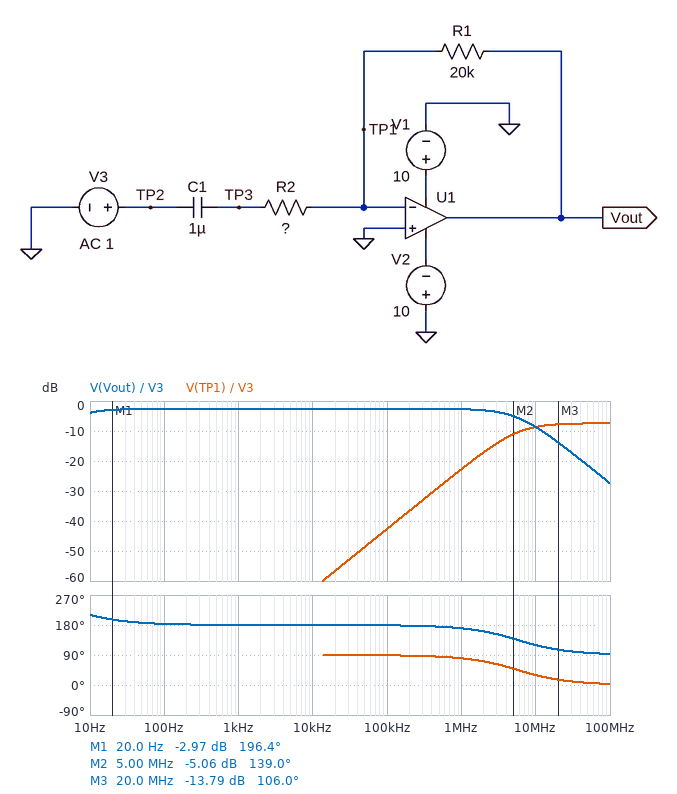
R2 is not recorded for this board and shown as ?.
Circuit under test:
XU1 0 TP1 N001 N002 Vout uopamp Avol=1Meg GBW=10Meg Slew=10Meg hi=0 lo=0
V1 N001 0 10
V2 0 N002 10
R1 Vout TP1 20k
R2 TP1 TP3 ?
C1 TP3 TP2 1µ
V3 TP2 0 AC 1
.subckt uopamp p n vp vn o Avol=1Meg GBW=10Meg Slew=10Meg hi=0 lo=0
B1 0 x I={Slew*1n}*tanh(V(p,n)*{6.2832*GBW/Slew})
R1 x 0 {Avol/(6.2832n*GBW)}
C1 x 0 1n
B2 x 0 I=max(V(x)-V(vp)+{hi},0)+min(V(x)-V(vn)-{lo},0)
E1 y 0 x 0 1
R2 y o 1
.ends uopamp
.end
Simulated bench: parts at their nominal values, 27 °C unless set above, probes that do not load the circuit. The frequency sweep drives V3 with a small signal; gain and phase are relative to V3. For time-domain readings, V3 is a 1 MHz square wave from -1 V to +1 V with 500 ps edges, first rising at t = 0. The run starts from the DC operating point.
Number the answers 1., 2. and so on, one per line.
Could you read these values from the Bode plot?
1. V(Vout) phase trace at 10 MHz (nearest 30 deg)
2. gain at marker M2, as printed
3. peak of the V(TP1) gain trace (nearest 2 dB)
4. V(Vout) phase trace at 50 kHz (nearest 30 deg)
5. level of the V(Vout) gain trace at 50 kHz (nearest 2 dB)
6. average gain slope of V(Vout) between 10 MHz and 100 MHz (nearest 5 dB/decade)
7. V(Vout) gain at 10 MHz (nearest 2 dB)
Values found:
1. 120 deg
2. -5.06 dB
3. -8 dB
4. 180 deg
5. -2 dB
6. -20 dB/decade
7. -8 dB
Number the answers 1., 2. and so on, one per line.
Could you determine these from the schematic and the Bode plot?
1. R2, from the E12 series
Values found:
1. 27 kΩ
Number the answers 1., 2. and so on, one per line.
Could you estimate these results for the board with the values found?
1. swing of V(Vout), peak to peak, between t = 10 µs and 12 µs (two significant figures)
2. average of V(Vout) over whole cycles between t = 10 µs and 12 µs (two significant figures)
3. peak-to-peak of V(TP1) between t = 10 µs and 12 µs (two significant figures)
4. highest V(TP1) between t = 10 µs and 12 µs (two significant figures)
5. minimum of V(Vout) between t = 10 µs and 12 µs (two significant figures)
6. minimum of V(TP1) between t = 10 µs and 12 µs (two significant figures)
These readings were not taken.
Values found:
1. 1.5 V
2. -740 mV
3. 1.7 V
4. 850 mV
5. -1.5 V
6. -850 mV
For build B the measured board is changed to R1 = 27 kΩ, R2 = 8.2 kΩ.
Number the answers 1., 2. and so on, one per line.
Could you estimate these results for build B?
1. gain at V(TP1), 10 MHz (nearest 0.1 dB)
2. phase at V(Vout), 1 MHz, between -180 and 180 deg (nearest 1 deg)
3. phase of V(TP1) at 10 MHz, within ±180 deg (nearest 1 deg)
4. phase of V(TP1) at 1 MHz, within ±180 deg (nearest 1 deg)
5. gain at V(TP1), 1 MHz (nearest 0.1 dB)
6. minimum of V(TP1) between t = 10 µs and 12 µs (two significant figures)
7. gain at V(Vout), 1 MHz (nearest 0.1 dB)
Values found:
1. -2.5 dB
2. 157 deg
3. 13 deg
4. 67 deg
5. -10.4 dB
6. -1.3 V
7. 9.6 dB
